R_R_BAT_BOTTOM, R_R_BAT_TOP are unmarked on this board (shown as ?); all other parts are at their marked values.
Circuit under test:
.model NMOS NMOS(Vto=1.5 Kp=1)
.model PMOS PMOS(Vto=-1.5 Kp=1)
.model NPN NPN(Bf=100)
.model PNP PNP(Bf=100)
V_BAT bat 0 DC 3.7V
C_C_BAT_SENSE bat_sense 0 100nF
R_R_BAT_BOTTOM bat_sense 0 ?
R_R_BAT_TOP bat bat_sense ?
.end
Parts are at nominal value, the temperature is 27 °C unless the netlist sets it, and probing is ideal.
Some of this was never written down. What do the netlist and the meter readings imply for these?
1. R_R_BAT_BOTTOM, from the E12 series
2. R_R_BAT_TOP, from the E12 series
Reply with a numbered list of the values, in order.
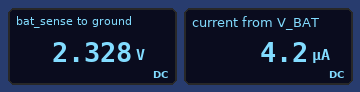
1. 560 kΩ
2. 330 kΩ
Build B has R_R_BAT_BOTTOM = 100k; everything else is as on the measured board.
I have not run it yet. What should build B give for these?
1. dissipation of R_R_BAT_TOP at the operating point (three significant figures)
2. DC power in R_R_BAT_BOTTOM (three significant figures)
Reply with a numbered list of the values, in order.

1. 24.4 µW
2. 7.40 µW
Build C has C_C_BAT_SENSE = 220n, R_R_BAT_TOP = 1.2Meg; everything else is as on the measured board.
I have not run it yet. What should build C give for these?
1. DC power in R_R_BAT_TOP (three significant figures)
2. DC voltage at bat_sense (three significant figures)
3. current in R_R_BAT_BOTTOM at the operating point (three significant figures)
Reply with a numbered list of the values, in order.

1. 5.30 µW
2. 1.18 V
3. 2.10 µA
